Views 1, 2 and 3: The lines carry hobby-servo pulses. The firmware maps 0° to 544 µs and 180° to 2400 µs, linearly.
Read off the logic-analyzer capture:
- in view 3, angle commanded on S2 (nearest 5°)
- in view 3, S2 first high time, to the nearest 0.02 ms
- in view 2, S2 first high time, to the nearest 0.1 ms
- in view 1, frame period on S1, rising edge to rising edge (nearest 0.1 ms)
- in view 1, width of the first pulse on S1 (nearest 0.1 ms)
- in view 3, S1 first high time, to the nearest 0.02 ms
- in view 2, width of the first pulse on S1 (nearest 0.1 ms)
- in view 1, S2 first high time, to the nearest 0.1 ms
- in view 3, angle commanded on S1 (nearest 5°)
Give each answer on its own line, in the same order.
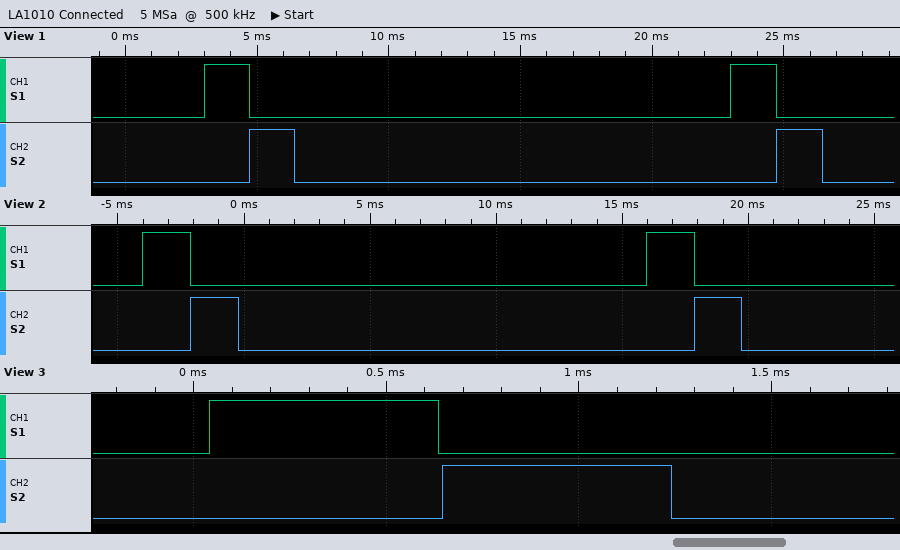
5°
0.60 ms
1.9 ms
20.0 ms
1.7 ms
0.60 ms
1.9 ms
1.7 ms
5°
